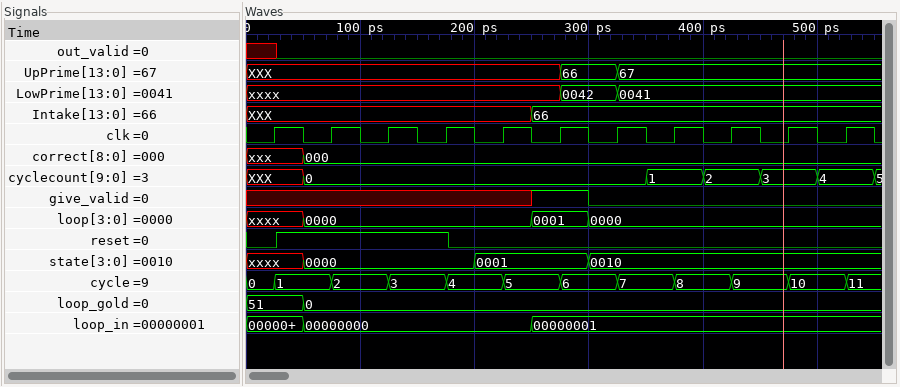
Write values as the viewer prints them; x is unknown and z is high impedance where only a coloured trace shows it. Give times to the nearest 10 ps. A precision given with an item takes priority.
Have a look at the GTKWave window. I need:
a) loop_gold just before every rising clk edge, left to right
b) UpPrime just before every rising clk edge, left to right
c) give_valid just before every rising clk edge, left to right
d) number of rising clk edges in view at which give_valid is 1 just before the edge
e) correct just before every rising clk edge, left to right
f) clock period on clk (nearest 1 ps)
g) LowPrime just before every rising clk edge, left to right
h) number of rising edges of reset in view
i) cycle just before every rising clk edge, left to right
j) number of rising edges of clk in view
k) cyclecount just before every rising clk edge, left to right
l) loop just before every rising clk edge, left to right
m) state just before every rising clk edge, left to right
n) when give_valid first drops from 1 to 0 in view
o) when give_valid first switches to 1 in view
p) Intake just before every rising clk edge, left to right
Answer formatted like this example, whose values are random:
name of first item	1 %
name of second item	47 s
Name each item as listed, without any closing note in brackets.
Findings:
loop_gold just before every rising clk edge, left to right	51, 0, 0, 0, 0, 0, 0, 0, 0, 0, 0
UpPrime just before every rising clk edge, left to right	XXX, XXX, XXX, XXX, XXX, XXX, 66, 67, 67, 67, 67
give_valid just before every rising clk edge, left to right	x x x x x 1 0 0 0 0 0
number of rising clk edges in view at which give_valid is 1 just before the edge	1
correct just before every rising clk edge, left to right	xxx, 000, 000, 000, 000, 000, 000, 000, 000, 000, 000
clock period on clk	50 ps
LowPrime just before every rising clk edge, left to right	xxxx, xxxx, xxxx, xxxx, xxxx, xxxx, 0042, 0041, 0041, 0041, 0041
number of rising edges of reset in view	1
cycle just before every rising clk edge, left to right	0, 1, 2, 3, 4, 5, 6, 7, 8, 9, 10
number of rising edges of clk in view	11
cyclecount just before every rising clk edge, left to right	XXX, 0, 0, 0, 0, 0, 0, 1, 2, 3, 4
loop just before every rising clk edge, left to right	xxxx, 0000, 0000, 0000, 0000, 0001, 0000, 0000, 0000, 0000, 0000
state just before every rising clk edge, left to right	xxxx, 0000, 0000, 0000, 0001, 0001, 0010, 0010, 0010, 0010, 0010
when give_valid first drops from 1 to 0 in view	300 ps
when give_valid first switches to 1 in view	250 ps
Intake just before every rising clk edge, left to right	XXX, XXX, XXX, XXX, XXX, 66, 66, 66, 66, 66, 66
